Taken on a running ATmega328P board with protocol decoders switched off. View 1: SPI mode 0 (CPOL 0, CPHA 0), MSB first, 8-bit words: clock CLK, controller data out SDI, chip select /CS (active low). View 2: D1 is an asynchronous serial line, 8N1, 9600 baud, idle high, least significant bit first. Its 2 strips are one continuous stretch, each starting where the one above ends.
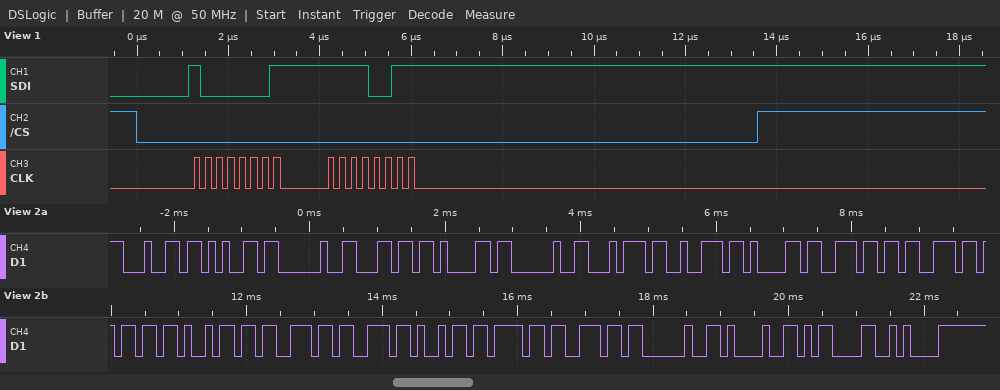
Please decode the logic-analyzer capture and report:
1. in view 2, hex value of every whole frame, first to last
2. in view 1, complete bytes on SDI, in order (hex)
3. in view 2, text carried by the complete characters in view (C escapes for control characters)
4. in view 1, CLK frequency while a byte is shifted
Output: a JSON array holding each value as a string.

["64 65 20 6C 61 20 74 72 61 6E 73 6D 69 73 73 69 6F 6E 20 21 0D 0A", "81 F3", "\"de la transmission !\\r\\n\"", "4 MHz"]
